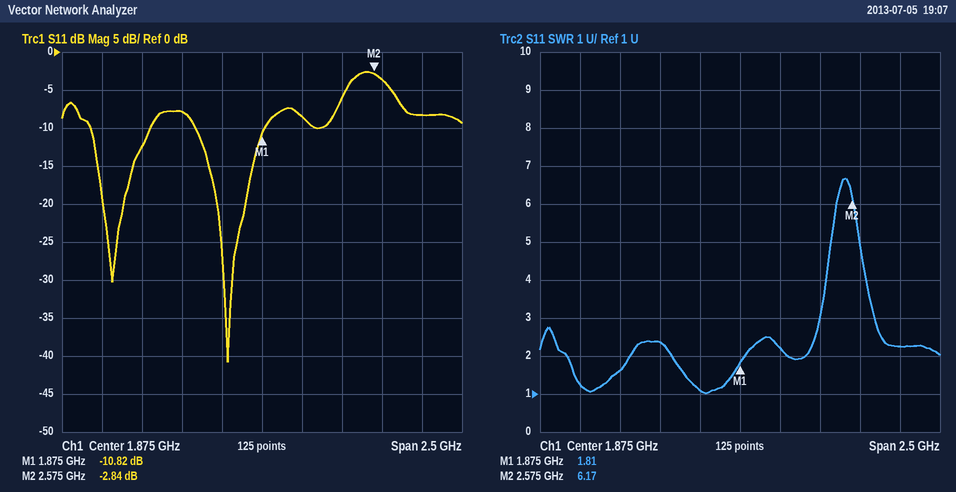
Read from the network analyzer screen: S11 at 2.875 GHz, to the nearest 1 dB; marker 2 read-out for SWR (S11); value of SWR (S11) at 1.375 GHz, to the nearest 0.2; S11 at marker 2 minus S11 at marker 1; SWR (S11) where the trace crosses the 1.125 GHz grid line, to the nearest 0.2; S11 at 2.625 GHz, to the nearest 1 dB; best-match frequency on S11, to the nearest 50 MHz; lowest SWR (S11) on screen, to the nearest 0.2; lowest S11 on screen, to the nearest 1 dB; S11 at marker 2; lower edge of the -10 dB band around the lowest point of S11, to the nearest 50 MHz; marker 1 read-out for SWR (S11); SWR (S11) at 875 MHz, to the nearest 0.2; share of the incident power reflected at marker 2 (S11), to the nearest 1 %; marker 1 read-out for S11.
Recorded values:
-8 dB
6.17
2.4
7.98 dB
1.6
-4 dB
1.65 GHz
1.0
-41 dB
-2.84 dB
1.45 GHz
1.81
1.2
52 %
-10.82 dB
